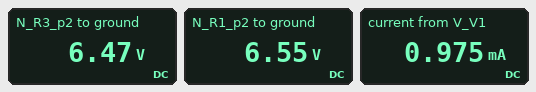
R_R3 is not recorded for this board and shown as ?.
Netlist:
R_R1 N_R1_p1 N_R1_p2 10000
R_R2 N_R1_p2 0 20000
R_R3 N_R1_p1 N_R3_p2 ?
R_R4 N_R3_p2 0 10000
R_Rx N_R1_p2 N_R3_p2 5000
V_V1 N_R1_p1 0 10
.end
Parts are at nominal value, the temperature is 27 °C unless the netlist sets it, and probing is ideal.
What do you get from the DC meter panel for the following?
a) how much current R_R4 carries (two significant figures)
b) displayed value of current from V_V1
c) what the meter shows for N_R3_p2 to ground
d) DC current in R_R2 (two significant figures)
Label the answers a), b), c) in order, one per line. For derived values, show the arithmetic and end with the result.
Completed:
a) (6.47 V) / 10 kΩ = 650 µA
b) 0.975 mA
c) 6.47 V
d) (6.55 V) / 20 kΩ = 330 µA
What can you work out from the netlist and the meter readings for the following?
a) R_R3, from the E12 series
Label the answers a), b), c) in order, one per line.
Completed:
a) 5.6 kΩ
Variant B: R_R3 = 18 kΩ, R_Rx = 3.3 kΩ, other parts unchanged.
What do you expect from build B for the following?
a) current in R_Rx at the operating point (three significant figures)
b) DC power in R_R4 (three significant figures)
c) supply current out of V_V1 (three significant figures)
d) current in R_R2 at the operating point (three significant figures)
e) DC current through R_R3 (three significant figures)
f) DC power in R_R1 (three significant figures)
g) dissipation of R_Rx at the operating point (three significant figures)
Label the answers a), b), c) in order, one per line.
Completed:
a) 189 µA
b) 2.29 mW
c) 749 µA
d) 270 µA
e) 290 µA
f) 2.11 mW
g) 118 µW
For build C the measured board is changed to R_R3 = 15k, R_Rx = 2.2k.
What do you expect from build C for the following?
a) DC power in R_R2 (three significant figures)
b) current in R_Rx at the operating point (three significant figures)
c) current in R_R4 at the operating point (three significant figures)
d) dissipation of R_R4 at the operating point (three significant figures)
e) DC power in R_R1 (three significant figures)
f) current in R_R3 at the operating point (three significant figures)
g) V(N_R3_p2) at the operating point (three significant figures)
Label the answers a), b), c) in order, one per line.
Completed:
a) 1.50 mW
b) 179 µA
c) 508 µA
d) 2.58 mW
e) 2.05 mW
f) 328 µA
g) 5.08 V
